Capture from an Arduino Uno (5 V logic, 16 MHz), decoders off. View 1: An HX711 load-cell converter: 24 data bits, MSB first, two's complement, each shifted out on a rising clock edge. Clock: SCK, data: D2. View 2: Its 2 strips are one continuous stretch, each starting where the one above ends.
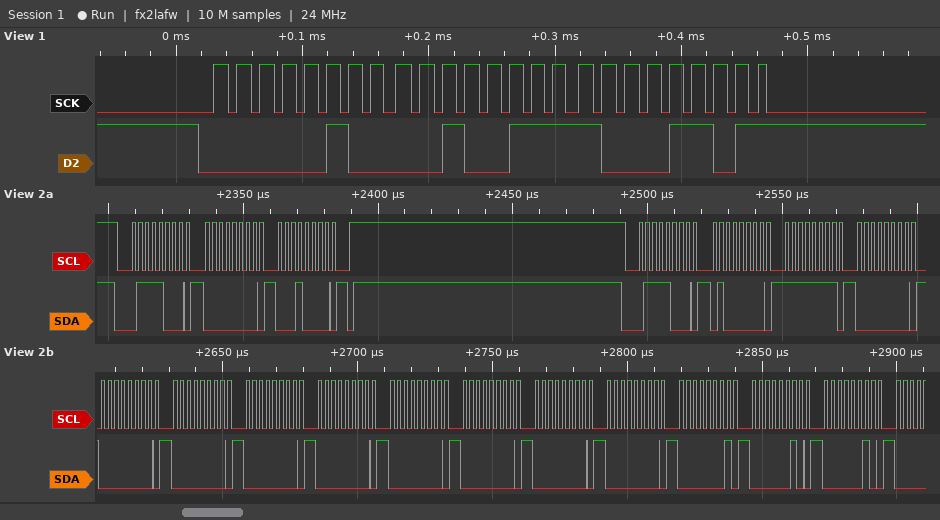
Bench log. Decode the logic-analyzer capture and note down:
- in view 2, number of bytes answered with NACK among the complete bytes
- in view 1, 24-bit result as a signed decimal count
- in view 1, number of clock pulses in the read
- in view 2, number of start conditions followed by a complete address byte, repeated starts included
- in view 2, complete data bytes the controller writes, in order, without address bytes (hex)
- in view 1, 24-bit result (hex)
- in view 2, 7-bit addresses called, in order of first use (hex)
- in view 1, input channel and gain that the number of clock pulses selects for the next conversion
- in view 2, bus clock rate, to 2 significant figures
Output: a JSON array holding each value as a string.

["0", "272269", "25", "2", "00 10 40 FF 00 00 00 00 00 00 00 00 00 01 02 02", "0x04278D", "0x3C", "channel A, gain 128", "400 kHz"]
